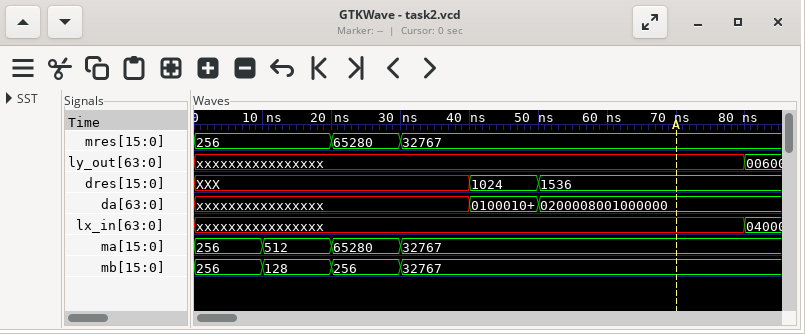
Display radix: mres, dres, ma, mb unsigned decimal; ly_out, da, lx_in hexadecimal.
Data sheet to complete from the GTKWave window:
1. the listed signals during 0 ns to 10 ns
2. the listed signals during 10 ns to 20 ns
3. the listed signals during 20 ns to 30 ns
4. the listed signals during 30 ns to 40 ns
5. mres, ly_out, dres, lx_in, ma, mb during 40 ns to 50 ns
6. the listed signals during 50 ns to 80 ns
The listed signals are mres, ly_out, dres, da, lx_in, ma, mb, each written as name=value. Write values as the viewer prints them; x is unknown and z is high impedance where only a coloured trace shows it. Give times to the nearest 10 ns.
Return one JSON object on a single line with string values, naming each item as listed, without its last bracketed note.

{"the listed signals during 0 ns to 10 ns": "mres=256, ly_out=xxxxxxxxxxxxxxxx, dres=XXX, da=xxxxxxxxxxxxxxxx, lx_in=xxxxxxxxxxxxxxxx, ma=256, mb=256", "the listed signals during 10 ns to 20 ns": "mres=256, ly_out=xxxxxxxxxxxxxxxx, dres=XXX, da=xxxxxxxxxxxxxxxx, lx_in=xxxxxxxxxxxxxxxx, ma=512, mb=128", "the listed signals during 20 ns to 30 ns": "mres=65280, ly_out=xxxxxxxxxxxxxxxx, dres=XXX, da=xxxxxxxxxxxxxxxx, lx_in=xxxxxxxxxxxxxxxx, ma=65280, mb=256", "the listed signals during 30 ns to 40 ns": "mres=32767, ly_out=xxxxxxxxxxxxxxxx, dres=XXX, da=xxxxxxxxxxxxxxxx, lx_in=xxxxxxxxxxxxxxxx, ma=32767, mb=32767", "mres, ly_out, dres, lx_in, ma, mb during 40 ns to 50 ns": "mres=32767, ly_out=xxxxxxxxxxxxxxxx, dres=1024, lx_in=xxxxxxxxxxxxxxxx, ma=32767, mb=32767", "the listed signals during 50 ns to 80 ns": "mres=32767, ly_out=xxxxxxxxxxxxxxxx, dres=1536, da=0200008001000000, lx_in=xxxxxxxxxxxxxxxx, ma=32767, mb=32767"}
